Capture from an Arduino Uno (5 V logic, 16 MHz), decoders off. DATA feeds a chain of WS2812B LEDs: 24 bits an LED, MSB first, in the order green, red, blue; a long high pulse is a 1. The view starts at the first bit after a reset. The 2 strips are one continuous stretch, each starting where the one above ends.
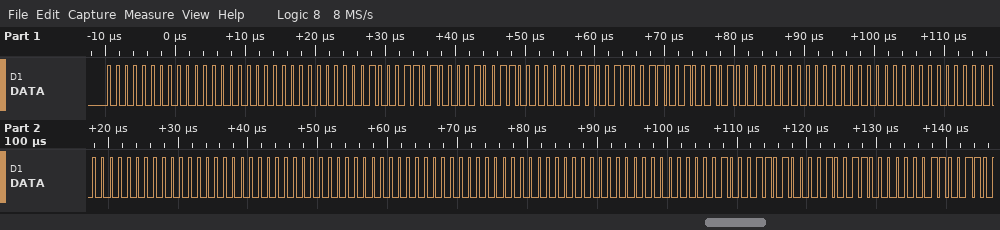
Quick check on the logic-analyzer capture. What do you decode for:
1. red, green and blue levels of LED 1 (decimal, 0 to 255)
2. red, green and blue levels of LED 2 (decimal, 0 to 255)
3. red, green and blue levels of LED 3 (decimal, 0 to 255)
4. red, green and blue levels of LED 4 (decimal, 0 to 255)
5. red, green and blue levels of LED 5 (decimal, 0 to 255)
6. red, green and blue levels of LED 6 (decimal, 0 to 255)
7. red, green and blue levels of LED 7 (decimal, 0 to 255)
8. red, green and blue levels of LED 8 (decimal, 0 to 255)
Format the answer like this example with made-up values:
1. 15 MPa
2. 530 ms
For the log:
1. 0, 0, 0
2. 52, 2, 38
3. 51, 3, 37
4. 0, 0, 0
5. 0, 0, 0
6. 0, 0, 0
7. 0, 0, 0
8. 52, 2, 38
